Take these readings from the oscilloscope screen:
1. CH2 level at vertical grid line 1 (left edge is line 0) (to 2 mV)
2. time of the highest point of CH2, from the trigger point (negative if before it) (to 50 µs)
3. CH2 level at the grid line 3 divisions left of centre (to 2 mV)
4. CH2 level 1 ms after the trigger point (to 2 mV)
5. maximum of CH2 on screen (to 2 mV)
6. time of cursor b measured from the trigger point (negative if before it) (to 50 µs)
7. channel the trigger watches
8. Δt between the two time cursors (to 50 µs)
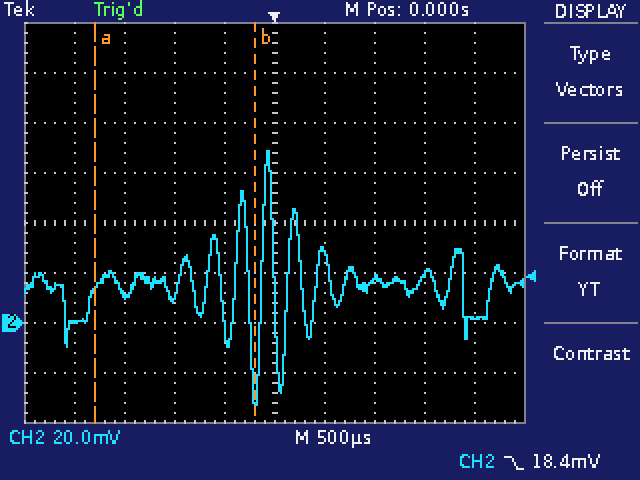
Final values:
0 mV
-50 µs
12 mV
18 mV
68 mV
-200 µs
CH2
1.60 ms
